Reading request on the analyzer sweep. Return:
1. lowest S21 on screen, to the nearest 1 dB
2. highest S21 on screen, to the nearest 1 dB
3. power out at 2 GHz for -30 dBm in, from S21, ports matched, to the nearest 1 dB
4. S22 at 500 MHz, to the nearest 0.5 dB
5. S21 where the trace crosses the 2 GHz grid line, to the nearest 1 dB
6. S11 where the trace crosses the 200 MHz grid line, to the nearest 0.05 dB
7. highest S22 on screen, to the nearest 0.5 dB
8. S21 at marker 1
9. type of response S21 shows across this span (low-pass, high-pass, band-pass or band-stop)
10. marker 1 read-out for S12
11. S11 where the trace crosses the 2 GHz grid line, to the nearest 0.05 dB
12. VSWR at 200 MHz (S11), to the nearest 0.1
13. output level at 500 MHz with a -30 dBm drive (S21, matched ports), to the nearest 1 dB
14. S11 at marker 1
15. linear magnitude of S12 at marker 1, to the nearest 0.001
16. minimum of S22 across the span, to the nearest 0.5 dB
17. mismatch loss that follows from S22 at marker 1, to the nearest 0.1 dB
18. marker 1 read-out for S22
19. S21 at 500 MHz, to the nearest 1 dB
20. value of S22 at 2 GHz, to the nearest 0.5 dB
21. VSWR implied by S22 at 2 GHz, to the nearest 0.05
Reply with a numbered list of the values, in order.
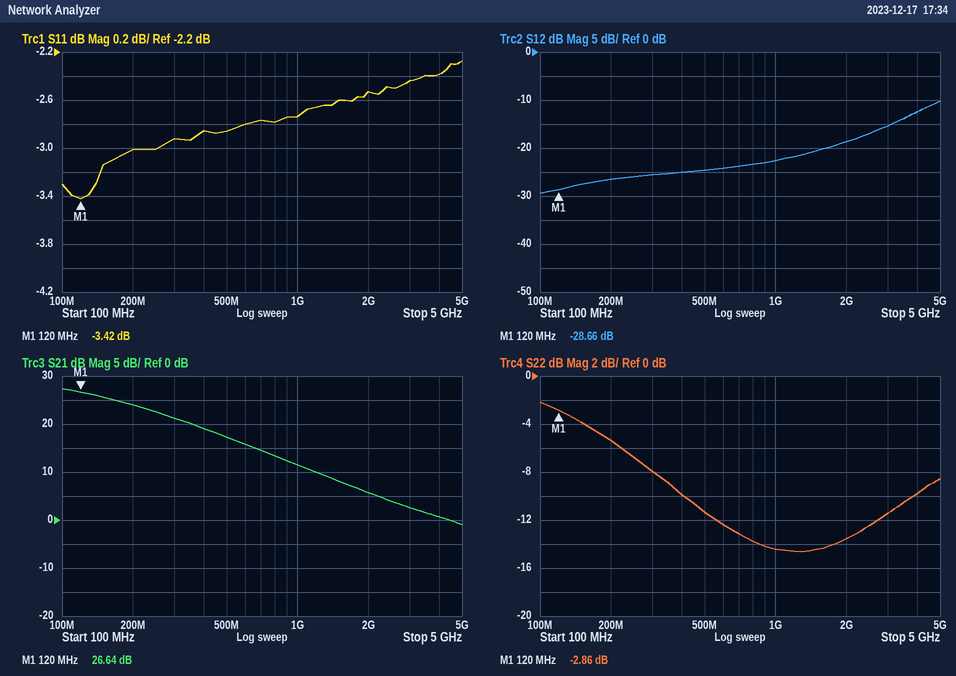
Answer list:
1. -1 dB
2. 27 dB
3. -24 dBm
4. -11.5 dB
5. 6 dB
6. -3.00 dB
7. -2.0 dB
8. 26.64 dB
9. low-pass
10. -28.66 dB
11. -2.55 dB
12. 5.8
13. -13 dBm
14. -3.42 dB
15. 0.037
16. -14.5 dB
17. 3.2 dB
18. -2.86 dB
19. 17 dB
20. -13.5 dB
21. 1.55
